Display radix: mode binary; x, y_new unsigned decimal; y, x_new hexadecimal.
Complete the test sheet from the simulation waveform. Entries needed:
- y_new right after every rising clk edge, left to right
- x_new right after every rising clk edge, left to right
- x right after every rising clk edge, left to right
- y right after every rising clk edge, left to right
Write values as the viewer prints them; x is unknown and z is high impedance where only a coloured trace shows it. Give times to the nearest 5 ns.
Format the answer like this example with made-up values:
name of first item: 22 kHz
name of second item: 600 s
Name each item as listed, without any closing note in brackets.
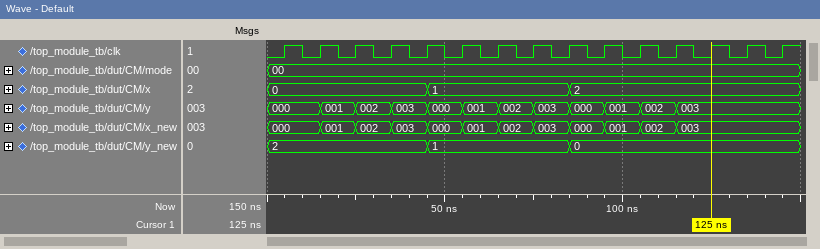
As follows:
y_new right after every rising clk edge, left to right: 2, 2, 2, 2, 1, 1, 1, 1, 0, 0, 0, 0, 0, 0, 0
x_new right after every rising clk edge, left to right: 000, 001, 002, 003, 000, 001, 002, 003, 000, 001, 002, 003, 003, 003, 003
x right after every rising clk edge, left to right: 0, 0, 0, 0, 1, 1, 1, 1, 2, 2, 2, 2, 2, 2, 2
y right after every rising clk edge, left to right: 000, 001, 002, 003, 000, 001, 002, 003, 000, 001, 002, 003, 003, 003, 003
